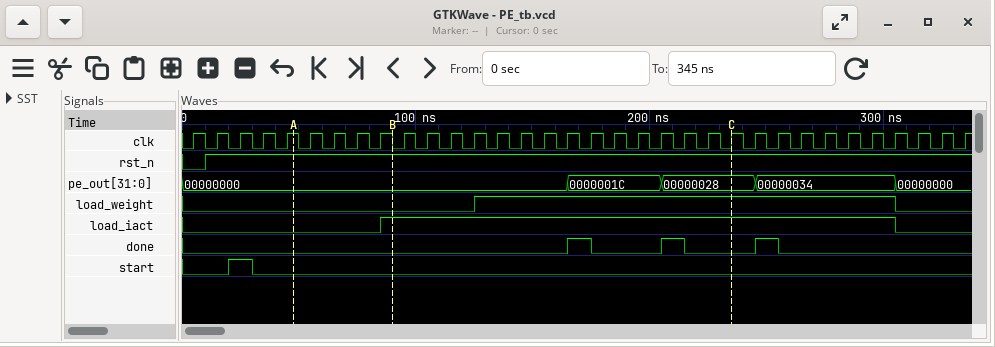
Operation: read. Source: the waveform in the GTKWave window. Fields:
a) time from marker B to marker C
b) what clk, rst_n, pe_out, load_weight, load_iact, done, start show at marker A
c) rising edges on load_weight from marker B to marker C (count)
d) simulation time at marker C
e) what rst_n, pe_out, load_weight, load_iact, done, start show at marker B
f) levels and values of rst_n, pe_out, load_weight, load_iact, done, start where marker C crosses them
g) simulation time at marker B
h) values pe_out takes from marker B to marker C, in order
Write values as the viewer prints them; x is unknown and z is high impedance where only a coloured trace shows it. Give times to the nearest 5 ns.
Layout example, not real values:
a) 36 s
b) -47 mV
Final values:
a) 145 ns
b) clk=1, rst_n=1, pe_out=00000000, load_weight=0, load_iact=0, done=0, start=0
c) 1
d) 235 ns
e) rst_n=1, pe_out=00000000, load_weight=0, load_iact=1, done=0, start=0
f) rst_n=1, pe_out=00000028, load_weight=1, load_iact=1, done=0, start=0
g) 90 ns
h) 00000000, 0000001C, 00000028
